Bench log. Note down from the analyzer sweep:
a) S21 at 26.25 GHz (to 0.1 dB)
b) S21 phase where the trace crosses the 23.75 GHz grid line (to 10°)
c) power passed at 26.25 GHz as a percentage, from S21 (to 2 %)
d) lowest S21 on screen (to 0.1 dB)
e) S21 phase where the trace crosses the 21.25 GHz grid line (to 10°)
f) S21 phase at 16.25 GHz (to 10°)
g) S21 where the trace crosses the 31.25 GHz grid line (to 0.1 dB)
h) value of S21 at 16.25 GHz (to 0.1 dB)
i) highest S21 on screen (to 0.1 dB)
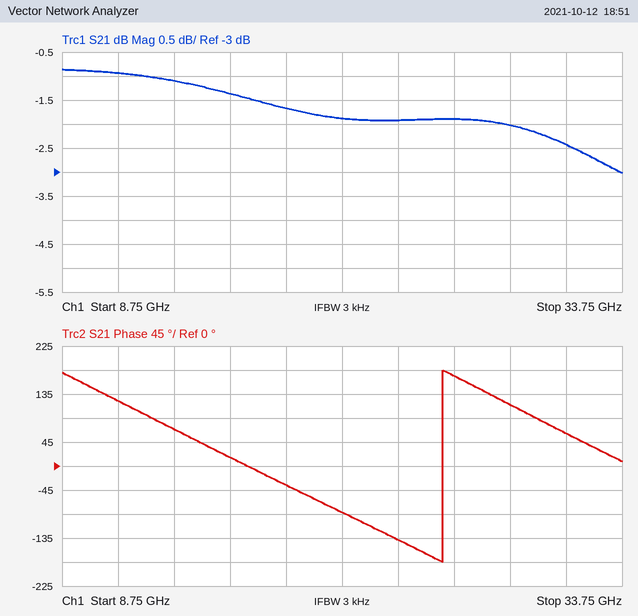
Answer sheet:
-1.9 dB
-140°
64 %
-3.0 dB
-90°
20°
-2.4 dB
-1.4 dB
-0.9 dB
